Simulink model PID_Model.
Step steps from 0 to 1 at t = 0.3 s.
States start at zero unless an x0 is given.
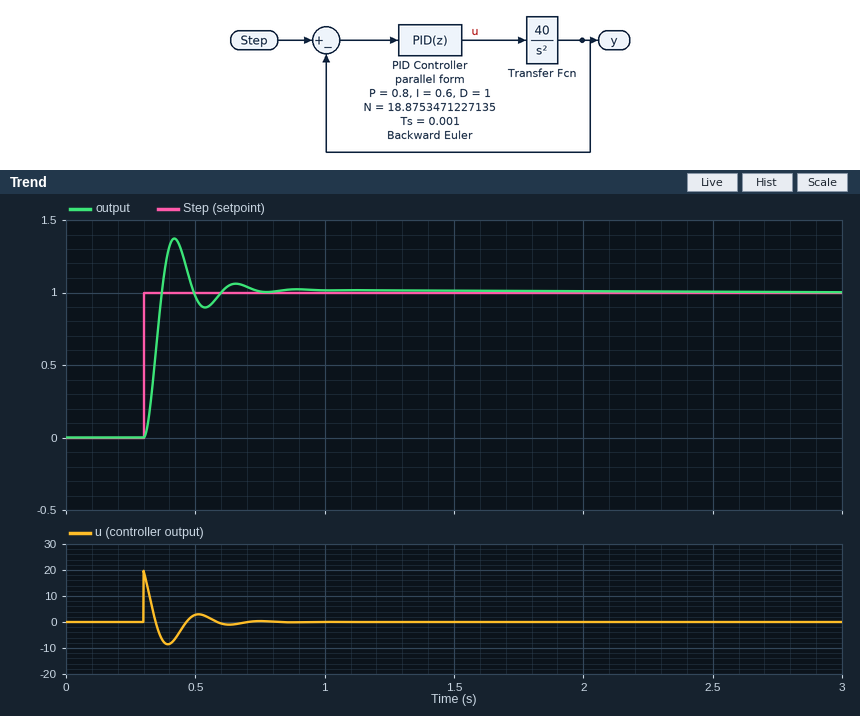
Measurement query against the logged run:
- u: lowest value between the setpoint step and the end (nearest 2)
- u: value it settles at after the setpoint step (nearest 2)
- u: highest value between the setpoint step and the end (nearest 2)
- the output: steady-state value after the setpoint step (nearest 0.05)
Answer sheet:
-8
0
20
1.00
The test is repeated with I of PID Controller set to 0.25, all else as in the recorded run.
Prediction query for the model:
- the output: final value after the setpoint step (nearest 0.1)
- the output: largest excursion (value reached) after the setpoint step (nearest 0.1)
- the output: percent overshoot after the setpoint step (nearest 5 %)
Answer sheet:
1.0
1.4
35 %
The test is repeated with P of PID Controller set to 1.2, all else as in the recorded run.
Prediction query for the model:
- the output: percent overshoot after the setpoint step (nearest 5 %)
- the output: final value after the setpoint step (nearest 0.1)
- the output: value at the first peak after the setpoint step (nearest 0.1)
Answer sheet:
40 %
1.0
1.4
